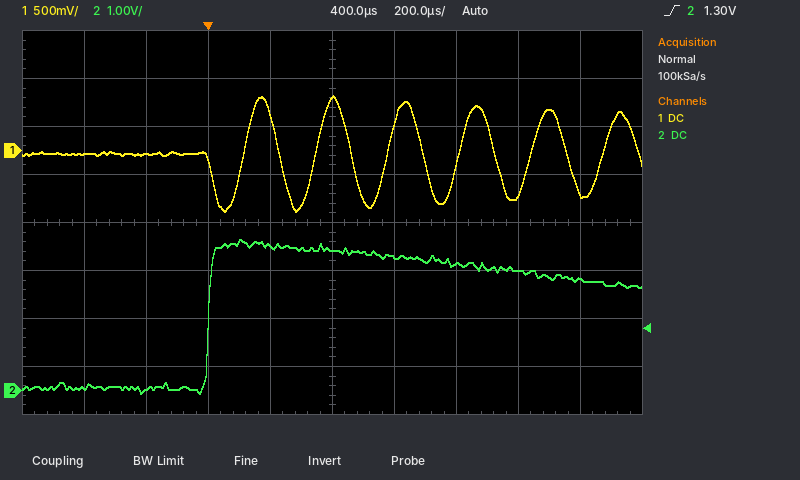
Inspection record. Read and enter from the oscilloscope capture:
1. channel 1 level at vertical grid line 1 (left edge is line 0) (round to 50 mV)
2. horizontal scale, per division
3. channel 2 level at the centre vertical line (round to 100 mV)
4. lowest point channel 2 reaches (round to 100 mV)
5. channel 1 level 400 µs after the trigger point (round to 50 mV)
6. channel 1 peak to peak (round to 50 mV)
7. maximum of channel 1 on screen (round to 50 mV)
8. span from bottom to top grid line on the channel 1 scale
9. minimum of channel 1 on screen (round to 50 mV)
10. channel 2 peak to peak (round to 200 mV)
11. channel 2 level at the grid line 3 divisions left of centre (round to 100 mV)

-50 mV
200 µs
2.9 V
-100 mV
550 mV
1.20 V
550 mV
4 V
-650 mV
3.2 V
0.0 V
